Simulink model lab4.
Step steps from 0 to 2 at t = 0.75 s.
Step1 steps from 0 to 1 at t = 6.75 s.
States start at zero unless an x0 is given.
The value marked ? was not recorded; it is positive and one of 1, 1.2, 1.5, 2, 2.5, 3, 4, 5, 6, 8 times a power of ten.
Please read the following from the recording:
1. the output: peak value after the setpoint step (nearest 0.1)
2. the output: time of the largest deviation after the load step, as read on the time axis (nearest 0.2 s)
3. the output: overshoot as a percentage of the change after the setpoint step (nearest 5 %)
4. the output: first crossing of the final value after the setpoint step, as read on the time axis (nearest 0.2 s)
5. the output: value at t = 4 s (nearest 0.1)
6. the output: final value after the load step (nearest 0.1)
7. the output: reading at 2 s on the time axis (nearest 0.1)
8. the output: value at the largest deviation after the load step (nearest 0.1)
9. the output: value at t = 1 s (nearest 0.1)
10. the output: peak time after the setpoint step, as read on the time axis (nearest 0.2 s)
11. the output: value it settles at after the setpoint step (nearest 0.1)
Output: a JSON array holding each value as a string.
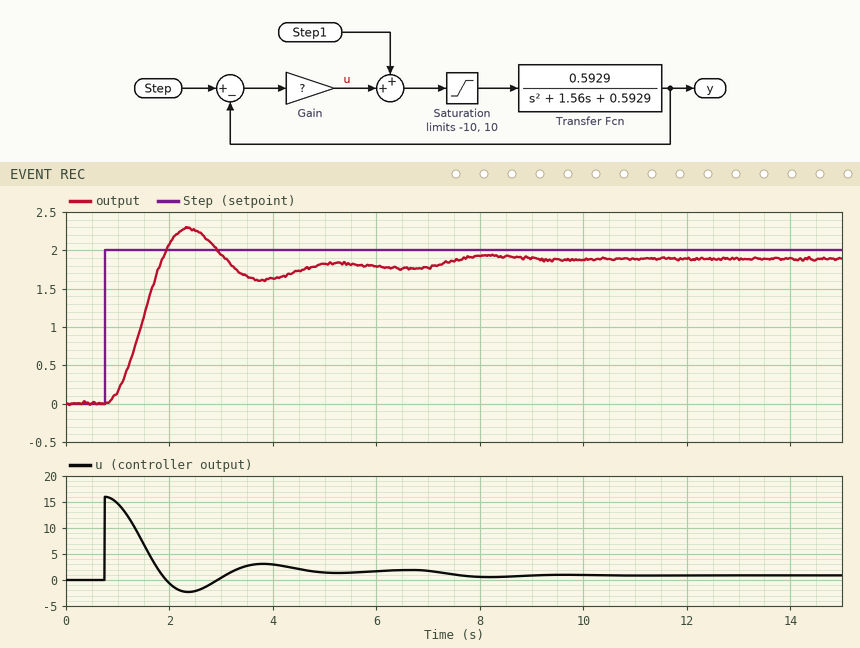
["2.3", "8.2 s", "30 %", "1.8 s", "1.6", "1.9", "2.1", "1.9", "0.2", "2.4 s", "1.8"]
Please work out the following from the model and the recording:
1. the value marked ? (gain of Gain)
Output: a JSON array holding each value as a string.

["8"]
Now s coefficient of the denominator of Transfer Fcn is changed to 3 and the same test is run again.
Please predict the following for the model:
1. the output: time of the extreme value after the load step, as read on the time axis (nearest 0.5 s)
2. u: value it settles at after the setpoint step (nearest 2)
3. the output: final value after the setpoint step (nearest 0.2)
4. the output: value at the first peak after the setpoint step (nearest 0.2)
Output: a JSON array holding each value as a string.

["8.5 s", "2", "1.8", "1.8"]
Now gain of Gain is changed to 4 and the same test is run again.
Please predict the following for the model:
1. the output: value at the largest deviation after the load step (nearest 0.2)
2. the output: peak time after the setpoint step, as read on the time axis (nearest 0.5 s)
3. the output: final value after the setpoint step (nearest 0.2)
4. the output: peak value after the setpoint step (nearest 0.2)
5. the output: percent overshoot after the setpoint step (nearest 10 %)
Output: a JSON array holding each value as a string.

["1.8", "3.0 s", "1.6", "2.0", "20 %"]
